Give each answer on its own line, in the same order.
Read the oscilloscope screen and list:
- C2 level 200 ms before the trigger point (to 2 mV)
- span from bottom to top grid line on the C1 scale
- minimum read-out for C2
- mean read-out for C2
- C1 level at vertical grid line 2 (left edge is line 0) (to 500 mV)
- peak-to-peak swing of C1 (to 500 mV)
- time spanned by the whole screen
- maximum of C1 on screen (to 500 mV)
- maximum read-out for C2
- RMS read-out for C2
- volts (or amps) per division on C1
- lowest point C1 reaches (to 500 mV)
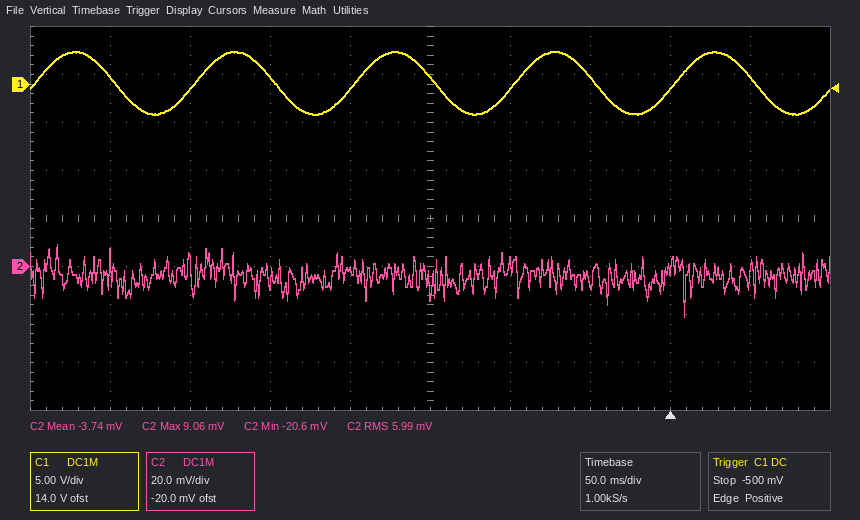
-2 mV
40 V
-20.6 mV
-3.74 mV
-500 mV
6.5 V
500 ms
3.5 V
9.06 mV
5.99 mV
5 V
-3.0 V
